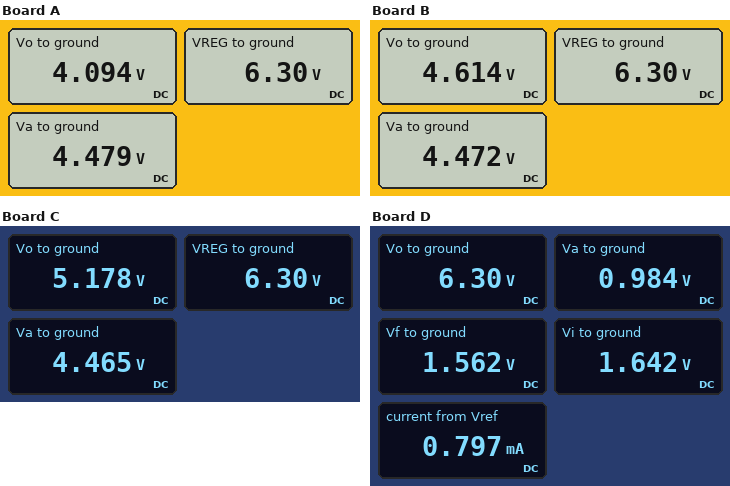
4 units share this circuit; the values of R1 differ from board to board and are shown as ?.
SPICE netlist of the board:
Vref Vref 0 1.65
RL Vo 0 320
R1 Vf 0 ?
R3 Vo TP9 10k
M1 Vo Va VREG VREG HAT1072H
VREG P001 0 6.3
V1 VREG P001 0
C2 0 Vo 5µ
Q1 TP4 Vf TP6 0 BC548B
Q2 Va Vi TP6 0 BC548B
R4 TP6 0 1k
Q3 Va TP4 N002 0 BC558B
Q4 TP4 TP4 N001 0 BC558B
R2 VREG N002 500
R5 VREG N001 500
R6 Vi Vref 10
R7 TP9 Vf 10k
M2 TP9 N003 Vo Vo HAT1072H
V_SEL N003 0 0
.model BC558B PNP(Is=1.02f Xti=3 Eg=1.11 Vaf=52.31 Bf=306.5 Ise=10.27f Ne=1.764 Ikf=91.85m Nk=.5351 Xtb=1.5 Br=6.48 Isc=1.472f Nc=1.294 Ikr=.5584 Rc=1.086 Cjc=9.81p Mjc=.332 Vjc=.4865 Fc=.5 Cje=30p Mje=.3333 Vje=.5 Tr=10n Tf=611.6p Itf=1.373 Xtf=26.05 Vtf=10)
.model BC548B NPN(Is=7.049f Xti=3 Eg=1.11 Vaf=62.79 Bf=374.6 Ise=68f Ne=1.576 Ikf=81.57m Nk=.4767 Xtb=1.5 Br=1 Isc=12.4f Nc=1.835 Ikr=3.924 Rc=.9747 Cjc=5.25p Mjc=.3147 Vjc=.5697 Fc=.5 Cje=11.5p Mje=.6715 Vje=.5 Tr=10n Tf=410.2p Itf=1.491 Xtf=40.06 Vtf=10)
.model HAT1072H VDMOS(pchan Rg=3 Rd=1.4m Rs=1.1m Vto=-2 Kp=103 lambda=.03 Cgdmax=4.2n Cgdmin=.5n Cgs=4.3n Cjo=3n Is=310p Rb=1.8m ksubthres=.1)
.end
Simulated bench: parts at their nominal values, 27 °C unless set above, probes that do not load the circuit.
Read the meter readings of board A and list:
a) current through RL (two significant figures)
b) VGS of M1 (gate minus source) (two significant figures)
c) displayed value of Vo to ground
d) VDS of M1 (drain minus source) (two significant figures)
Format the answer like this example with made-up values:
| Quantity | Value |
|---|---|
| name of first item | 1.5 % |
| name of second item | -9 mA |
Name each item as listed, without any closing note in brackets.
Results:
| Quantity | Value |
|---|---|
| current through RL | 13 mA |
| VGS of M1 (gate minus source) | -1.8 V |
| displayed value of Vo to ground | 4.094 V |
| VDS of M1 (drain minus source) | -2.2 V |
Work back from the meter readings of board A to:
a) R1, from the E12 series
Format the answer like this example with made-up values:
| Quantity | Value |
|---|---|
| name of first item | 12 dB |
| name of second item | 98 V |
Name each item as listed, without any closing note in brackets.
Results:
| Quantity | Value |
|---|---|
| R1, from the E12 series | 6.8 kΩ |
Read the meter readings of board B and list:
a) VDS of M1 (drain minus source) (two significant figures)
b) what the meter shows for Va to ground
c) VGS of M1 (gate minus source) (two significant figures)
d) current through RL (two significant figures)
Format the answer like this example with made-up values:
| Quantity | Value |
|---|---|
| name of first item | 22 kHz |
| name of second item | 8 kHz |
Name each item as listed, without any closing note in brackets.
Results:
| Quantity | Value |
|---|---|
| VDS of M1 (drain minus source) | -1.7 V |
| what the meter shows for Va to ground | 4.472 V |
| VGS of M1 (gate minus source) | -1.8 V |
| current through RL | 14 mA |
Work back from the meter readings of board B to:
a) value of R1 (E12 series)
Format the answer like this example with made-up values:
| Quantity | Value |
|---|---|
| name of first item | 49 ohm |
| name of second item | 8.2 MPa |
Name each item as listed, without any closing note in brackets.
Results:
| Quantity | Value |
|---|---|
| value of R1 | 5.6 kΩ |
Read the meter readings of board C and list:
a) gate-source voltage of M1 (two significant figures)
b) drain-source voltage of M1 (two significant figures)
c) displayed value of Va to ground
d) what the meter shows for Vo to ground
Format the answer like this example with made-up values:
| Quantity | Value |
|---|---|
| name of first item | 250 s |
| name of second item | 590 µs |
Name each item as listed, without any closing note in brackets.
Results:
| Quantity | Value |
|---|---|
| gate-source voltage of M1 | -1.8 V |
| drain-source voltage of M1 | -1.1 V |
| displayed value of Va to ground | 4.465 V |
| what the meter shows for Vo to ground | 5.178 V |
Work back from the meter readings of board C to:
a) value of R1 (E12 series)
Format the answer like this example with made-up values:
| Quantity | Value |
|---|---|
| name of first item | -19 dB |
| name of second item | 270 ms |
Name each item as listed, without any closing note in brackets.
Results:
| Quantity | Value |
|---|---|
| value of R1 | 4.7 kΩ |
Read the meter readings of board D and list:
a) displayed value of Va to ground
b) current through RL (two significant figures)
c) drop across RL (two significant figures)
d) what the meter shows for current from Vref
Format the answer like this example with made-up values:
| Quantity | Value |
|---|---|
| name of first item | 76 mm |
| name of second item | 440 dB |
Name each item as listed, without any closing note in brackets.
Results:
| Quantity | Value |
|---|---|
| displayed value of Va to ground | 0.984 V |
| current through RL | 20 mA |
| drop across RL | 6.3 V |
| what the meter shows for current from Vref | 0.797 mA |
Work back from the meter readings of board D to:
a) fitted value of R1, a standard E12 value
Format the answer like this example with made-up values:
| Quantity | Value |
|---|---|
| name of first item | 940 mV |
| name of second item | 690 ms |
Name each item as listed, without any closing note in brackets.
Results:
| Quantity | Value |
|---|---|
| fitted value of R1, a standard E12 value | 3.3 kΩ |
